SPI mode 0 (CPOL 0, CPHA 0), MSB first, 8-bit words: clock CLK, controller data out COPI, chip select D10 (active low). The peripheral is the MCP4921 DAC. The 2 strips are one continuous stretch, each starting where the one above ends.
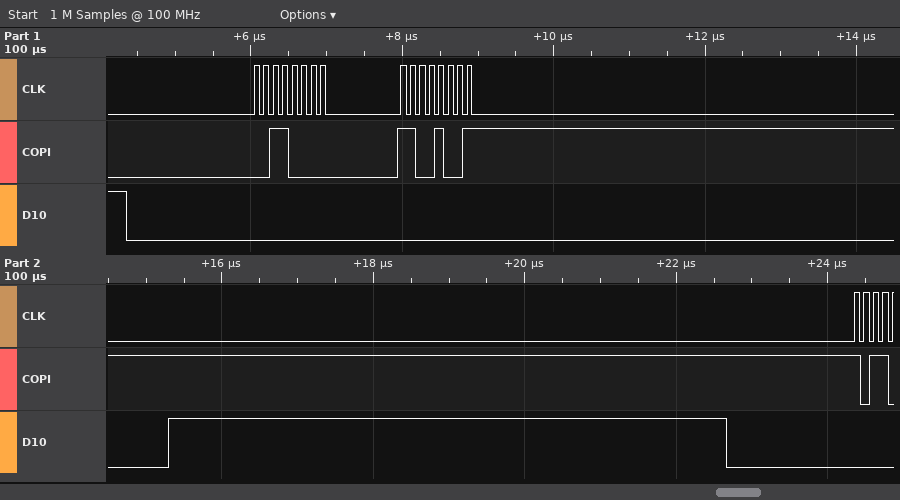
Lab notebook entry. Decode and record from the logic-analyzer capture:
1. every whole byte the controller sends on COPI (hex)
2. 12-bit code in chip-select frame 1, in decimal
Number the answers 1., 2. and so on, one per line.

1. 30 C9
2. 201
